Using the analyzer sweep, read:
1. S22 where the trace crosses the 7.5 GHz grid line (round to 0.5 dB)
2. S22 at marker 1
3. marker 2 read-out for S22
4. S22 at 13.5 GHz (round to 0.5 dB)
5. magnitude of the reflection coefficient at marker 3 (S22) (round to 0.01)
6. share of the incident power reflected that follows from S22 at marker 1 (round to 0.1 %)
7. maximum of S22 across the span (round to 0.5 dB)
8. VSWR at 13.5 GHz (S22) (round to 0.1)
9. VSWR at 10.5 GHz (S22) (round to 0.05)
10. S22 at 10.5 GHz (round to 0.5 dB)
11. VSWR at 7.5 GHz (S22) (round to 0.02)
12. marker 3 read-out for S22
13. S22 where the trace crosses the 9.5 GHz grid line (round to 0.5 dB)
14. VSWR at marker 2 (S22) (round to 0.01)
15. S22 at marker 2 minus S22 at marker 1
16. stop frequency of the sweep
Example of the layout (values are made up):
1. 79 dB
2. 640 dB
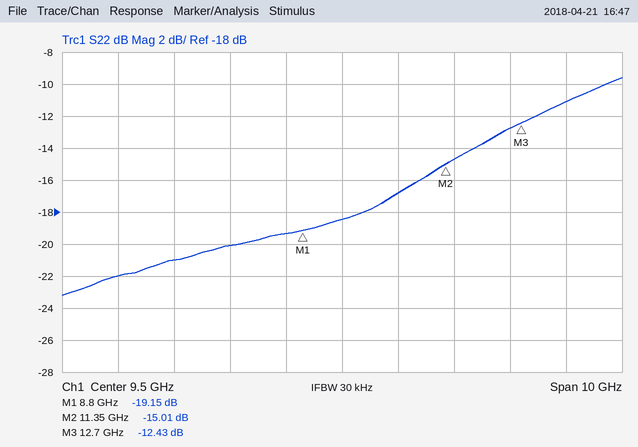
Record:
1. -20.0 dB
2. -19.15 dB
3. -15.01 dB
4. -11.0 dB
5. 0.24
6. 1.2 %
7. -9.5 dB
8. 1.8
9. 1.35
10. -17.0 dB
11. 1.22
12. -12.43 dB
13. -18.5 dB
14. 1.43
15. 4.14 dB
16. 14.5 GHz
